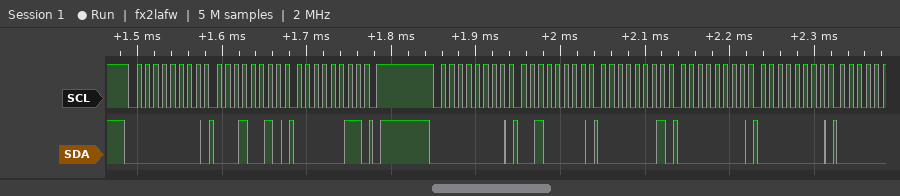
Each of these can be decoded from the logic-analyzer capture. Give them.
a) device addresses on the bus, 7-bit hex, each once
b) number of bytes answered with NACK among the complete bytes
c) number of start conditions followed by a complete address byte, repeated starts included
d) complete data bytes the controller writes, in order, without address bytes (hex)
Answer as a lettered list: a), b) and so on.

a) 0x00
b) 0
c) 2
d) 12 03 20 01 00 00
